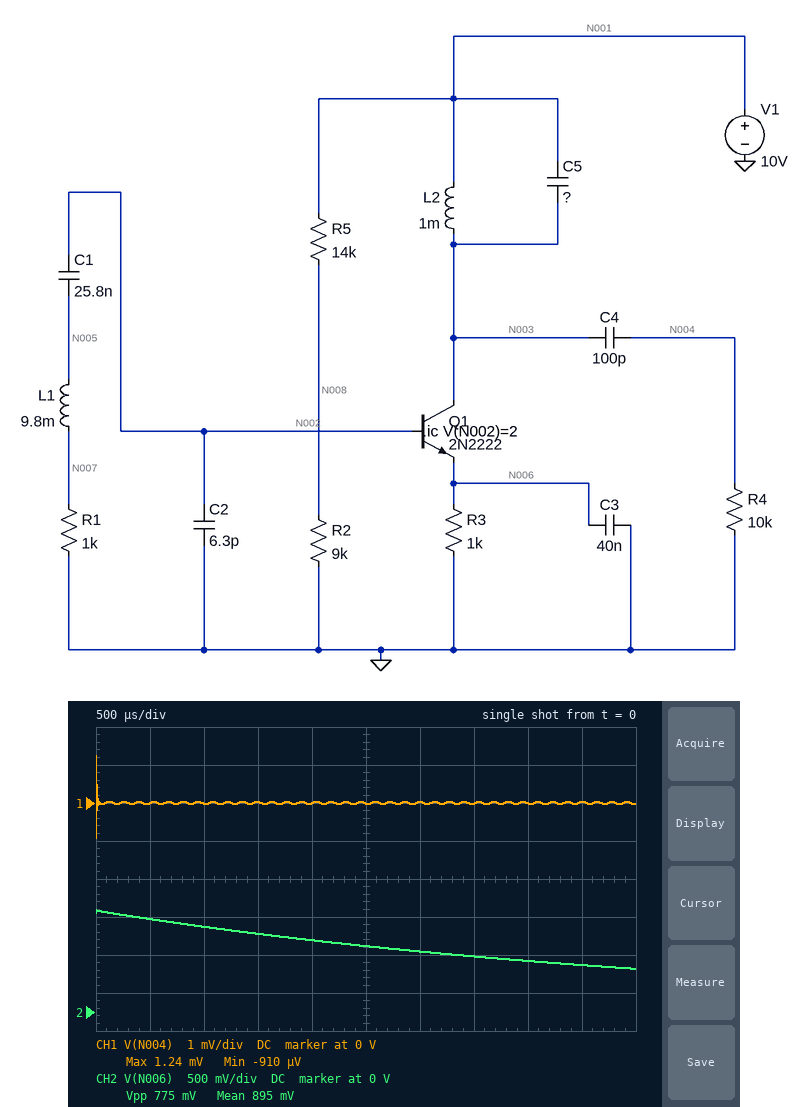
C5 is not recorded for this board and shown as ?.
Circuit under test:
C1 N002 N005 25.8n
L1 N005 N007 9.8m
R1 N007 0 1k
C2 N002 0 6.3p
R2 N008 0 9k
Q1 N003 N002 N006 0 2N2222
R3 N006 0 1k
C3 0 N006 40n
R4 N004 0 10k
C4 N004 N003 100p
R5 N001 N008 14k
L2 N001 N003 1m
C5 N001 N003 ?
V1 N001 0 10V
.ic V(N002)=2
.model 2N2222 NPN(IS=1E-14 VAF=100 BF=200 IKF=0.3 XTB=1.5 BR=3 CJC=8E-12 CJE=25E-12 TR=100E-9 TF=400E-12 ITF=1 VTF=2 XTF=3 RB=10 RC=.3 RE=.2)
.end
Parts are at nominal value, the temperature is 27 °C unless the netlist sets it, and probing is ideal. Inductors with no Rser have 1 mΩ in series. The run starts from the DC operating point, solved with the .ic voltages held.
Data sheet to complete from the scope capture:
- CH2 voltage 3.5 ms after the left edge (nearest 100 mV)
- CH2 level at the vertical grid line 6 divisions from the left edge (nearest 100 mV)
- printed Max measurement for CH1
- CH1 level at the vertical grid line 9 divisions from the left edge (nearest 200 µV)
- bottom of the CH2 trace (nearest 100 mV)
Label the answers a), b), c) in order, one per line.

a) 700 mV
b) 800 mV
c) 1.24 mV
d) 0 V
e) 600 mV
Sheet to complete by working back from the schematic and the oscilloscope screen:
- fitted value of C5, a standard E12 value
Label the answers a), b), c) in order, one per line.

a) 470 nF
